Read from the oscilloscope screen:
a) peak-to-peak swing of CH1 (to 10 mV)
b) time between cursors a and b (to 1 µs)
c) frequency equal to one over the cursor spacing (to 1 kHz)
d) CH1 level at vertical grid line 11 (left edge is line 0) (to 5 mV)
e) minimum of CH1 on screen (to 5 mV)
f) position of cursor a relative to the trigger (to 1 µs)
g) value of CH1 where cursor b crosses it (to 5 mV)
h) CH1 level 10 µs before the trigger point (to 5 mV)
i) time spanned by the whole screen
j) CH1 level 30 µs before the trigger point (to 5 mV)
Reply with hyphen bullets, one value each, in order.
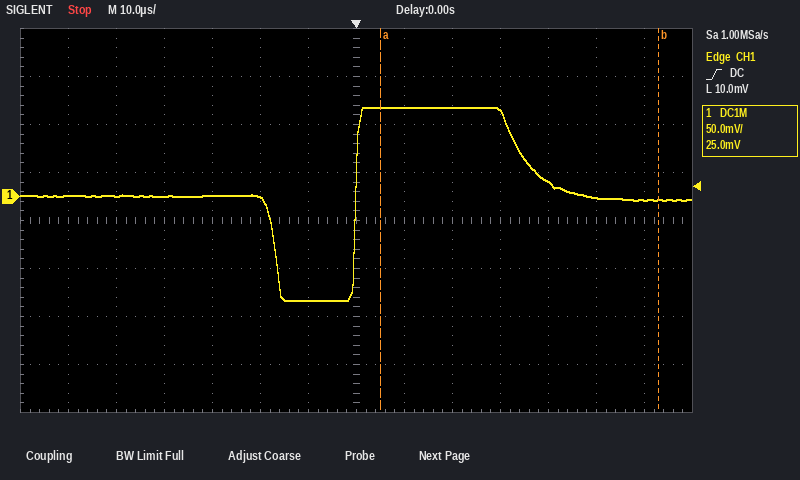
- 200 mV
- 58 µs
- 17 kHz
- 15 mV
- -110 mV
- +5 µs
- -5 mV
- -110 mV
- 140 µs
- 0 mV
